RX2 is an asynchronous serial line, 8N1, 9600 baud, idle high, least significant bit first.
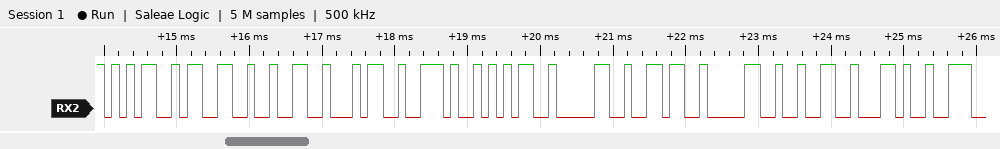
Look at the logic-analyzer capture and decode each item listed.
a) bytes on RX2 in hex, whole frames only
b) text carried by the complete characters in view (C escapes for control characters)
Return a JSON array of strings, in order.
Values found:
["0x35 0x33 0x32 0x34 0x2E 0x35 0x30 0x36 0x30 0x32 0x2C", "\"5324.50602,\""]
